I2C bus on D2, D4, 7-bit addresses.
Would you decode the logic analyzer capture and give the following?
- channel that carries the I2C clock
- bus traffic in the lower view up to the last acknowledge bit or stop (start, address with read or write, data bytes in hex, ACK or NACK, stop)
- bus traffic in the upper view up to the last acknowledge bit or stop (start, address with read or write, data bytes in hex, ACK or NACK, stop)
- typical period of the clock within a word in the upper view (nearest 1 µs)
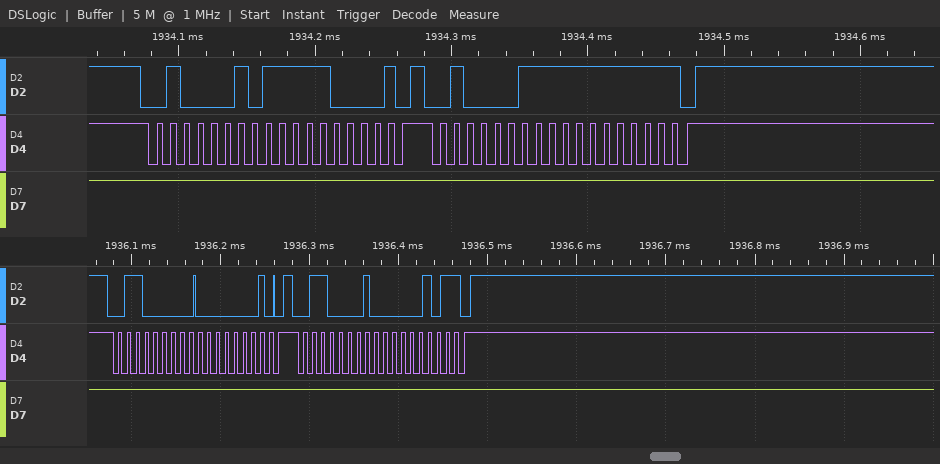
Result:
D4
start, address 30 write ACK, 01 ACK, stop, start, address 30 read ACK, 05 NACK, stop
start, address 21 write NACK, F0 NACK, stop, start, address 21 read NACK, FF NACK, stop
10 µs
